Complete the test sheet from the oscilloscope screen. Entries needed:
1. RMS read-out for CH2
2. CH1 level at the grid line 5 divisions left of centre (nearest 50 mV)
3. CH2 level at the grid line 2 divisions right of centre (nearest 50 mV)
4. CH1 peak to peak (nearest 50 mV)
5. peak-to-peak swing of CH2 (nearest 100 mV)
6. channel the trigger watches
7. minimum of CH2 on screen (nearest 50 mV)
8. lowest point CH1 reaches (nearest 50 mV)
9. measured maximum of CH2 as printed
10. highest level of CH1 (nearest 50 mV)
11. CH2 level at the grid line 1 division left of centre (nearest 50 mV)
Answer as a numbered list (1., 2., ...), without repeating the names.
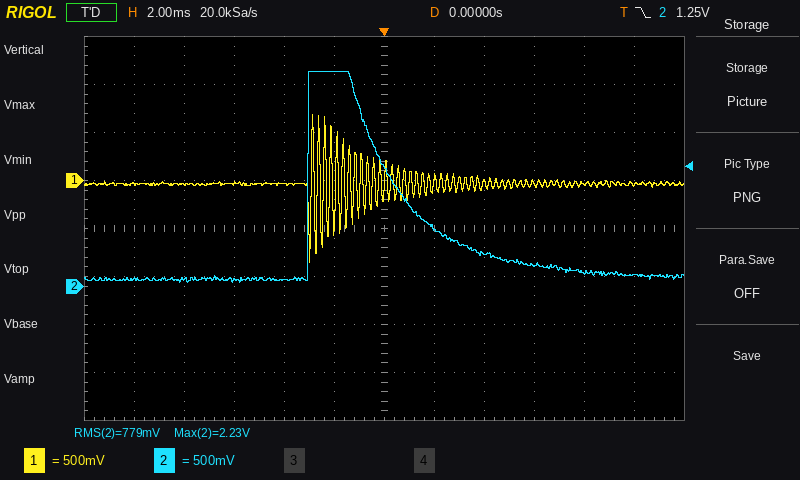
1. 779 mV
2. -50 mV
3. 350 mV
4. 1.55 V
5. 2.20 V
6. CH2
7. 50 mV
8. -850 mV
9. 2.23 V
10. 700 mV
11. 2.25 V
